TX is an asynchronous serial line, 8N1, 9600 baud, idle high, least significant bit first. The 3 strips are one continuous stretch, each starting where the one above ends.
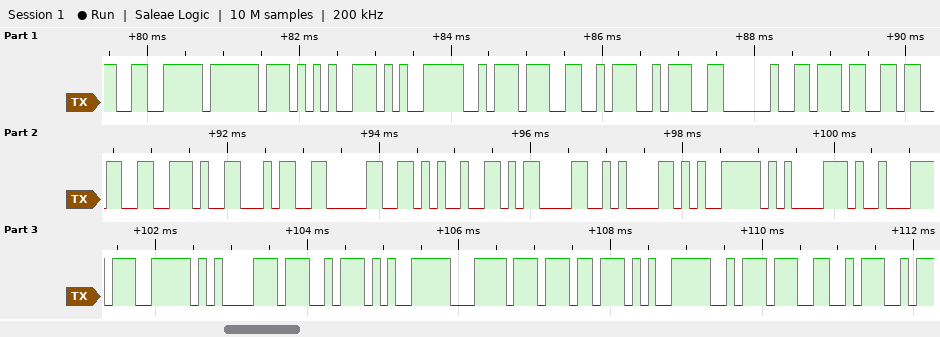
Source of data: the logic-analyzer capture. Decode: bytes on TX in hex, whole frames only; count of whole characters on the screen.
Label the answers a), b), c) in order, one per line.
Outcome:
a) E6 BF 95 E5 BA A6 3A 20 37 33 2E 34 30 25 0D 0A E5 85 89 E7 85 A7 E5 BC B7 E5 BA A6
b) 28
